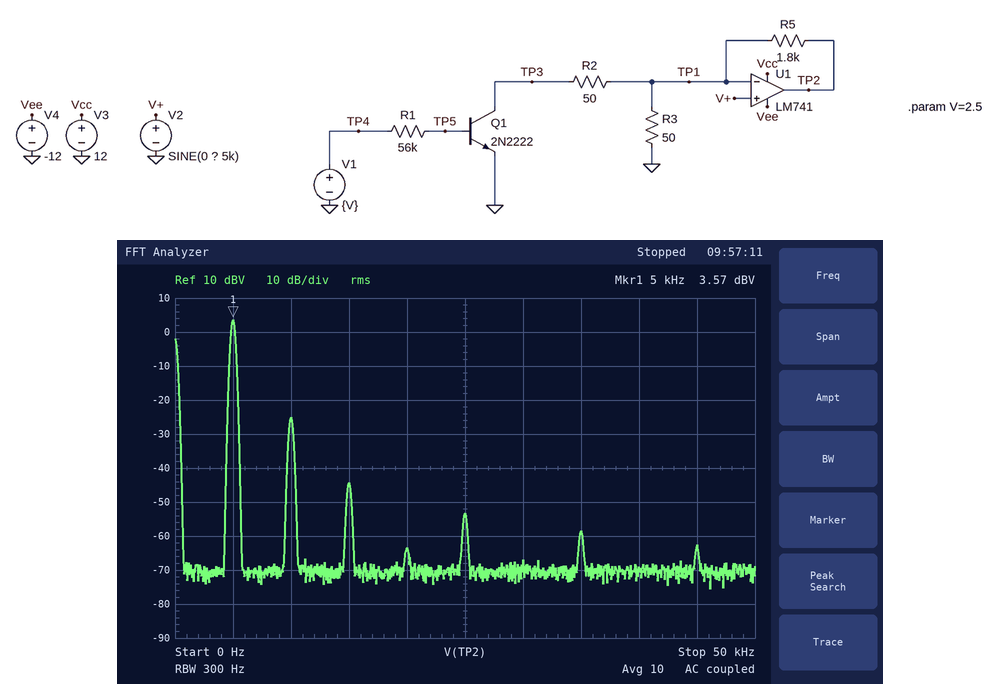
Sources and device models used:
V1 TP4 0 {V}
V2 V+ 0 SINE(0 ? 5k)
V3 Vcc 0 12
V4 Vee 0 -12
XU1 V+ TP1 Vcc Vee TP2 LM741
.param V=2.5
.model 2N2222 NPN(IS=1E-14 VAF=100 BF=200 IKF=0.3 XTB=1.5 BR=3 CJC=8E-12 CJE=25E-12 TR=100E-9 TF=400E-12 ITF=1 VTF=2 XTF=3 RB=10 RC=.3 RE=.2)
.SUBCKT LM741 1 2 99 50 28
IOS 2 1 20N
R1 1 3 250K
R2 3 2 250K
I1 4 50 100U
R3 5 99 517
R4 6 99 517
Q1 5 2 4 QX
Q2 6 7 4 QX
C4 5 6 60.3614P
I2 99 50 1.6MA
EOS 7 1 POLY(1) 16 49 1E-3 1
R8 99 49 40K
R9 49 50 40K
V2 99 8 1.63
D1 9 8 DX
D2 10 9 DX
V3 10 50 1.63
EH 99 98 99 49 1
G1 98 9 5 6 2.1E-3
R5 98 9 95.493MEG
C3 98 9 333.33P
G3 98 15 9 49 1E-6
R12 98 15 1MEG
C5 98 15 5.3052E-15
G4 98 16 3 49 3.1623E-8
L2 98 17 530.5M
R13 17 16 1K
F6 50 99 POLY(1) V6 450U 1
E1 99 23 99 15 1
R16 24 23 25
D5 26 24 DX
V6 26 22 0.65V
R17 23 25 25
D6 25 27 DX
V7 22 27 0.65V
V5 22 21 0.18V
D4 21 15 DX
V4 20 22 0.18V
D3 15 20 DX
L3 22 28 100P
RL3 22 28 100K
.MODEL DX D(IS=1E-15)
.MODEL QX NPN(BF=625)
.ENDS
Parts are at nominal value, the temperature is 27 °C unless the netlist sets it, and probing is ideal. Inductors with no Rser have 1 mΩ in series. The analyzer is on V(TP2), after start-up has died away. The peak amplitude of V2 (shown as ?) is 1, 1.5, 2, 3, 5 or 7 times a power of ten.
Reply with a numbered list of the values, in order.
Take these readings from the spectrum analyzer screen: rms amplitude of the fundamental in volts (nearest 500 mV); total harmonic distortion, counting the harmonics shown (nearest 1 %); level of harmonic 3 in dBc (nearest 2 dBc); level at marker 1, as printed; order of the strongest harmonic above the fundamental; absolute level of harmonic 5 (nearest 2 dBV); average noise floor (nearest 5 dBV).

1. 1.5 V
2. 4 %
3. -48 dBc
4. 3.57 dBV
5. 2
6. -54 dBV
7. -70 dBV
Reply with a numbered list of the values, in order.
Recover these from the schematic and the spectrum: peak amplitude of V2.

1. 50 mV
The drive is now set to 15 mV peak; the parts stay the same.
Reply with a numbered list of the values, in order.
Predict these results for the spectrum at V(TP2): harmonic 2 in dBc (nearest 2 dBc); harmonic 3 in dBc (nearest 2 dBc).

1. -38 dBc
2. -52 dBc
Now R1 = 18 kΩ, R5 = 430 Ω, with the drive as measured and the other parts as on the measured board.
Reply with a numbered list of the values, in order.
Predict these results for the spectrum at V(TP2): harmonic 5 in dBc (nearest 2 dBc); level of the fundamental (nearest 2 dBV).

1. -52 dBc
2. -6 dBV
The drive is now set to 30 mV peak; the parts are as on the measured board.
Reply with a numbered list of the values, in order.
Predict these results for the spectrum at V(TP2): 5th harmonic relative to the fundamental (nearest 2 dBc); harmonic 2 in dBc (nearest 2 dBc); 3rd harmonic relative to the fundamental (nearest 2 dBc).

1. -58 dBc
2. -32 dBc
3. -50 dBc
